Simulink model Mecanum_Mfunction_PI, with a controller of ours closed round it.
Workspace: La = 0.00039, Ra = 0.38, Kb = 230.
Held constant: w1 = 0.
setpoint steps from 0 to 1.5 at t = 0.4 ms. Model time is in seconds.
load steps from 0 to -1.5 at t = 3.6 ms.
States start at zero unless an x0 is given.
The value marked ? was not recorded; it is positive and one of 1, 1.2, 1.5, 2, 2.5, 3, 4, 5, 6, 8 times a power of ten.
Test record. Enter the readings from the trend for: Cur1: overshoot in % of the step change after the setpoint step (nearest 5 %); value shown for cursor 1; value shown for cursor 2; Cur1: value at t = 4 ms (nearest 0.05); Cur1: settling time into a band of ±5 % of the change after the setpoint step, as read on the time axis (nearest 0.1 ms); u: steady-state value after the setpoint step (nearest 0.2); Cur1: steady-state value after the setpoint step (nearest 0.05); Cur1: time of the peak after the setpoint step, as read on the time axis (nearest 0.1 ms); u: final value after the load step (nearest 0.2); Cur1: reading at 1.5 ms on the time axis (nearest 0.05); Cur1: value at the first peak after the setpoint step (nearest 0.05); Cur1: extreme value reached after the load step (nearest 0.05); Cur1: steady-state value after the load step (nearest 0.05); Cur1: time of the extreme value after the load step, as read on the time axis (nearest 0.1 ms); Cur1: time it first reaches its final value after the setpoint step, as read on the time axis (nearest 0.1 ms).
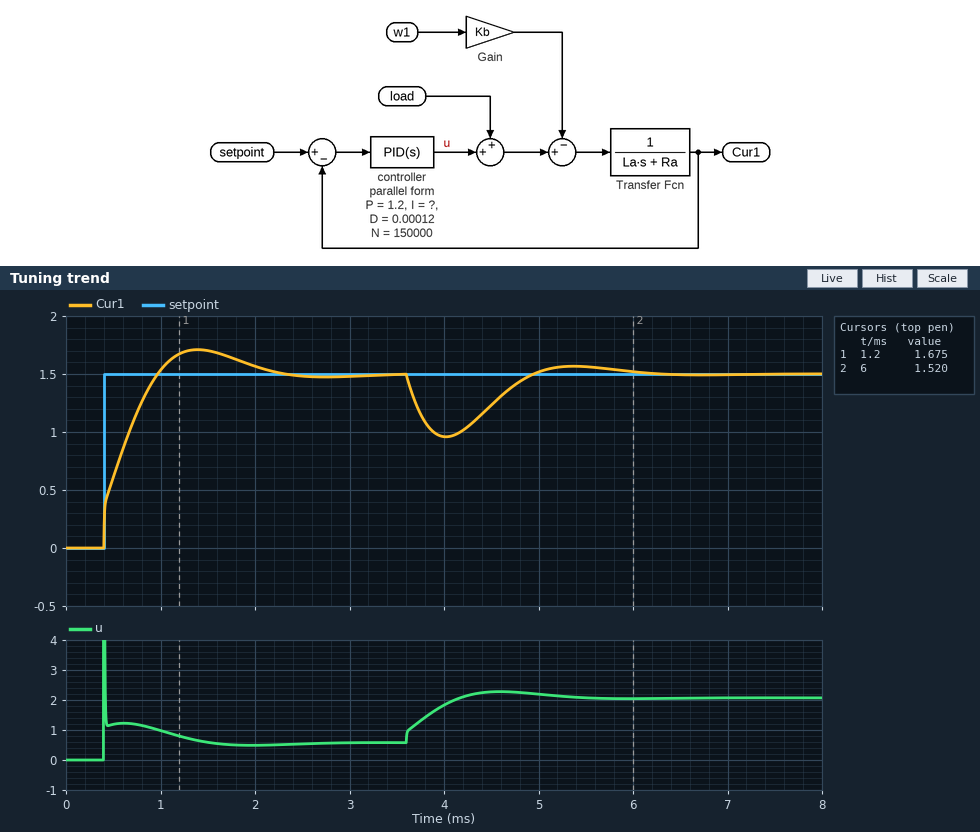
15 %
1.675
1.520
0.95
2.0 ms
0.6
1.50
1.4 ms
2.0
1.70
1.70
0.95
1.50
4.0 ms
1.0 ms
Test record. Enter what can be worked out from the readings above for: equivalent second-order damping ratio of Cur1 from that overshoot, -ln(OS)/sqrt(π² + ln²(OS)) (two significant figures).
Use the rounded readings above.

0.52
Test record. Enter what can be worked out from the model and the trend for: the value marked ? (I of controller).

4000
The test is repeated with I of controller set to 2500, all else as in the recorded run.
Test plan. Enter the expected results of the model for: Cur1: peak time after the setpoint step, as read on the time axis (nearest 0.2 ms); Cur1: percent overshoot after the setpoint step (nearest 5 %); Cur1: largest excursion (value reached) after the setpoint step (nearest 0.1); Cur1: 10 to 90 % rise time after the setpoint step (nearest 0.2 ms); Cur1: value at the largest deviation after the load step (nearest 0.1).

1.6 ms
10 %
1.6
0.6 ms
0.9
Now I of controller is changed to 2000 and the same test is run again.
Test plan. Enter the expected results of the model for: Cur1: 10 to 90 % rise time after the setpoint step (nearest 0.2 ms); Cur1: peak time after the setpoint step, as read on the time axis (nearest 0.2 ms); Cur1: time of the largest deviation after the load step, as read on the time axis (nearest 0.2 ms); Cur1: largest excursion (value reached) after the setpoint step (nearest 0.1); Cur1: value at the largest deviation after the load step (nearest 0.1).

0.6 ms
1.8 ms
4.2 ms
1.6
0.9
